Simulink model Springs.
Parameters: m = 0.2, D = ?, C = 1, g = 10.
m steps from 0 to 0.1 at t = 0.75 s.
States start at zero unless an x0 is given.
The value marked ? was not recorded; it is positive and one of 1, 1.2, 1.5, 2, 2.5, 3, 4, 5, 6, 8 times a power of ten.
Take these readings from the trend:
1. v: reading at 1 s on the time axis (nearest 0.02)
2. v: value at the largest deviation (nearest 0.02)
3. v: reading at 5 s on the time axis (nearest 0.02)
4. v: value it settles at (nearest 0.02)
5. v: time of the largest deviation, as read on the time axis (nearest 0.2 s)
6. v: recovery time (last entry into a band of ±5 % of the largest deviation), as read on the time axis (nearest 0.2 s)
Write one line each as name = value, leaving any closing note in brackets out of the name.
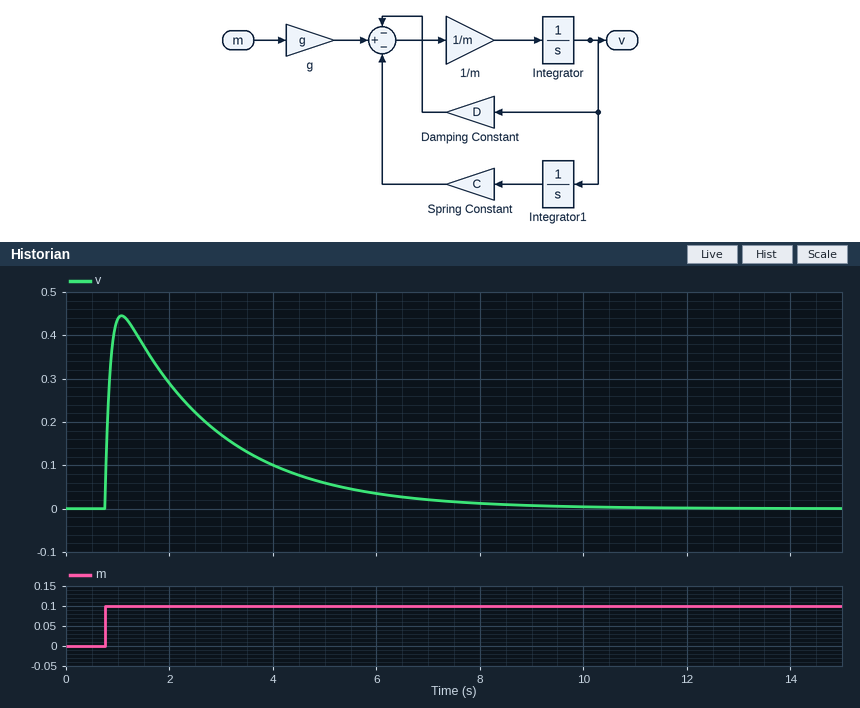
v: reading at 1 s on the time axis = 0.44
v: value at the largest deviation = 0.44
v: reading at 5 s on the time axis = 0.06
v: value it settles at = 0.00
v: time of the largest deviation, as read on the time axis = 1.0 s
v: recovery time (last entry into a band of ±5 % of the largest deviation), as read on the time axis = 6.8 s
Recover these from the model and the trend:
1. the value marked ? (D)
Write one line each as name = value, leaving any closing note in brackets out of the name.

the value marked ? = 2
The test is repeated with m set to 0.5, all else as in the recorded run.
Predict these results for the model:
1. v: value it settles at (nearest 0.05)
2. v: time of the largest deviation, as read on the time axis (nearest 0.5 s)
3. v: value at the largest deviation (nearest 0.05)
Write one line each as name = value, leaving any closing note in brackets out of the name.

v: value it settles at = 0.00
v: time of the largest deviation, as read on the time axis = 1.5 s
v: value at the largest deviation = 0.40
